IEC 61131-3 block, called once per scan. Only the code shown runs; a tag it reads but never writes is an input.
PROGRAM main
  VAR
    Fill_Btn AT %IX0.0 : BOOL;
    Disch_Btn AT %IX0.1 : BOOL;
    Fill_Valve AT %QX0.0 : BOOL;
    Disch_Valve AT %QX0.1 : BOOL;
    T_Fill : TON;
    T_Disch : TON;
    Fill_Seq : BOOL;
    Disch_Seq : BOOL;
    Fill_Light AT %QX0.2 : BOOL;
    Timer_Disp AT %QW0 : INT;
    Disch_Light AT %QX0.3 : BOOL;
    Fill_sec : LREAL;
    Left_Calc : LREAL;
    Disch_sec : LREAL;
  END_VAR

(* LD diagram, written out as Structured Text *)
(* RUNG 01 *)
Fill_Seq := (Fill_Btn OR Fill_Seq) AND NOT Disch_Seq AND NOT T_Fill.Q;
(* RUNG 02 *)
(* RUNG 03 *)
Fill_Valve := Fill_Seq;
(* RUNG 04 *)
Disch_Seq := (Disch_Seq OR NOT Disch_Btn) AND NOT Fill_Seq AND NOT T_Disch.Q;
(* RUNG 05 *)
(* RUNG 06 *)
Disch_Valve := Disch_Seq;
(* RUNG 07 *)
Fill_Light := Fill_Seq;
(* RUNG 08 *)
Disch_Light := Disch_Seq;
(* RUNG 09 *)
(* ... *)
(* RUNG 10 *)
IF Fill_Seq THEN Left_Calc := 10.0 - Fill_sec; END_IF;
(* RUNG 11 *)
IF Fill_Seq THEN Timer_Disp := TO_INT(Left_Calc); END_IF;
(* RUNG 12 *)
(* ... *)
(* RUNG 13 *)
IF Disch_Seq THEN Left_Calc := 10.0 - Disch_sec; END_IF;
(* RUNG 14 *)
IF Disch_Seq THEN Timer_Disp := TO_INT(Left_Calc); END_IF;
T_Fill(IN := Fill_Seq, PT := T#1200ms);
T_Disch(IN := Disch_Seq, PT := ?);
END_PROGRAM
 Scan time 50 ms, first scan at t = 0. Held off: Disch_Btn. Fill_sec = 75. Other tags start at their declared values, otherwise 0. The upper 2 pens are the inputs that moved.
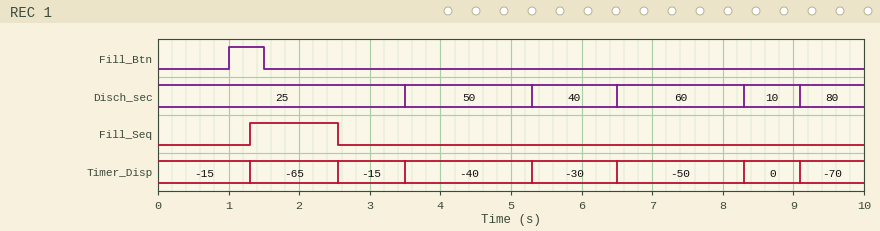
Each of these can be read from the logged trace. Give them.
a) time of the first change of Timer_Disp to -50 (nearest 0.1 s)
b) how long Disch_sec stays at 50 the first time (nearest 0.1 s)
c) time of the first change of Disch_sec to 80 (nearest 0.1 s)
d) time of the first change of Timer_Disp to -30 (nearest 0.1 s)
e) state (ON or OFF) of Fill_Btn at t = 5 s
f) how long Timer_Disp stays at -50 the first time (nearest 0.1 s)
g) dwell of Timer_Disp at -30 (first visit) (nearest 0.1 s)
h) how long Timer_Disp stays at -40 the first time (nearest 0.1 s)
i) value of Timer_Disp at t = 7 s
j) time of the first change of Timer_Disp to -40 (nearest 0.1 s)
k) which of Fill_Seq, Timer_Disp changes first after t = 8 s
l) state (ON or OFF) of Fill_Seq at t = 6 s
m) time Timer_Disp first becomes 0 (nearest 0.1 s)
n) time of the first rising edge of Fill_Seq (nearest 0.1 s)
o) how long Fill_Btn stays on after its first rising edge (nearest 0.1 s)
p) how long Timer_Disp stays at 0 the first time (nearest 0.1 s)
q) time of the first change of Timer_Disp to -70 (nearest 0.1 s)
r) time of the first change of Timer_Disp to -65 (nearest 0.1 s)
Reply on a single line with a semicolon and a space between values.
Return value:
6.5 s; 1.8 s; 9.1 s; 5.3 s; OFF; 1.8 s; 1.2 s; 1.8 s; -50; 3.5 s; Timer_Disp; OFF; 8.3 s; 1.3 s; 0.5 s; 0.8 s; 9.1 s; 1.3 s
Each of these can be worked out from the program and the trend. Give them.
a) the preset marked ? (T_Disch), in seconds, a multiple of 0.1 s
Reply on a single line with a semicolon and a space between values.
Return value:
1.2 s
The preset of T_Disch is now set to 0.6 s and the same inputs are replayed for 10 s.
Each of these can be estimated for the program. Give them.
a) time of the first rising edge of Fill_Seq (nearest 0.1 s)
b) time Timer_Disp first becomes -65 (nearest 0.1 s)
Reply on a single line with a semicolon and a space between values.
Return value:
1.4 s; 1.4 s
